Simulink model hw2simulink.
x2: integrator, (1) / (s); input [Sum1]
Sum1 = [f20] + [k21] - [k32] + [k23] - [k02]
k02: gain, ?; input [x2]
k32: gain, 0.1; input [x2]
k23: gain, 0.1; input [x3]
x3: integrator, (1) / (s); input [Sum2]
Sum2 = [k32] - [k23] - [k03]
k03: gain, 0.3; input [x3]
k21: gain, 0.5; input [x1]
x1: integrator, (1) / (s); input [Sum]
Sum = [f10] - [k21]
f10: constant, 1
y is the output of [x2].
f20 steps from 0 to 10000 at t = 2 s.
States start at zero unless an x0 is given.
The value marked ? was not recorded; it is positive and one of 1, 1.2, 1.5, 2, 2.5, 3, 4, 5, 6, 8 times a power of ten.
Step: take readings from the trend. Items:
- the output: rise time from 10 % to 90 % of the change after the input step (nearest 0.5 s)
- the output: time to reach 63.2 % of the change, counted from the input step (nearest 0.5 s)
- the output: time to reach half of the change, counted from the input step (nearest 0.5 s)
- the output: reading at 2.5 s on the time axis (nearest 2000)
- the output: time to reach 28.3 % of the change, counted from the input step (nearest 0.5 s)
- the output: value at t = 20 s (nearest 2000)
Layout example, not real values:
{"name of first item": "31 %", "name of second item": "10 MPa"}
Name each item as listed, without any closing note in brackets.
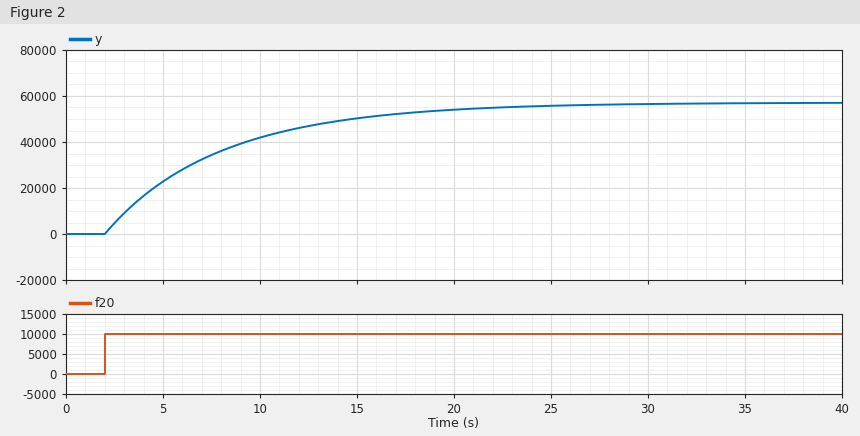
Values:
{"the output: rise time from 10 % to 90 % of the change after the input step": "13.5 s", "the output: time to reach 63.2 % of the change, counted from the input step": "6.0 s", "the output: time to reach half of the change, counted from the input step": "4.0 s", "the output: reading at 2.5 s on the time axis": "4000", "the output: time to reach 28.3 % of the change, counted from the input step": "2.0 s", "the output: value at t = 20 s": "54000"}
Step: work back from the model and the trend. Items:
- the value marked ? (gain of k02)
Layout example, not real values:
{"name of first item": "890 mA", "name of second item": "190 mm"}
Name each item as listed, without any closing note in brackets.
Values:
{"the value marked ?": "0.1"}
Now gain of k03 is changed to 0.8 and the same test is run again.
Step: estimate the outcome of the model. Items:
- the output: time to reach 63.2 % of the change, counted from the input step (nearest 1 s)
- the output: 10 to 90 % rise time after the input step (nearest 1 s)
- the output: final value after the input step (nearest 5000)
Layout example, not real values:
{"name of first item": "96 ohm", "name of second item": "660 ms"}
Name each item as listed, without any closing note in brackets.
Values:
{"the output: time to reach 63.2 % of the change, counted from the input step": "5 s", "the output: 10 to 90 % rise time after the input step": "12 s", "the output: final value after the input step": "55000"}
